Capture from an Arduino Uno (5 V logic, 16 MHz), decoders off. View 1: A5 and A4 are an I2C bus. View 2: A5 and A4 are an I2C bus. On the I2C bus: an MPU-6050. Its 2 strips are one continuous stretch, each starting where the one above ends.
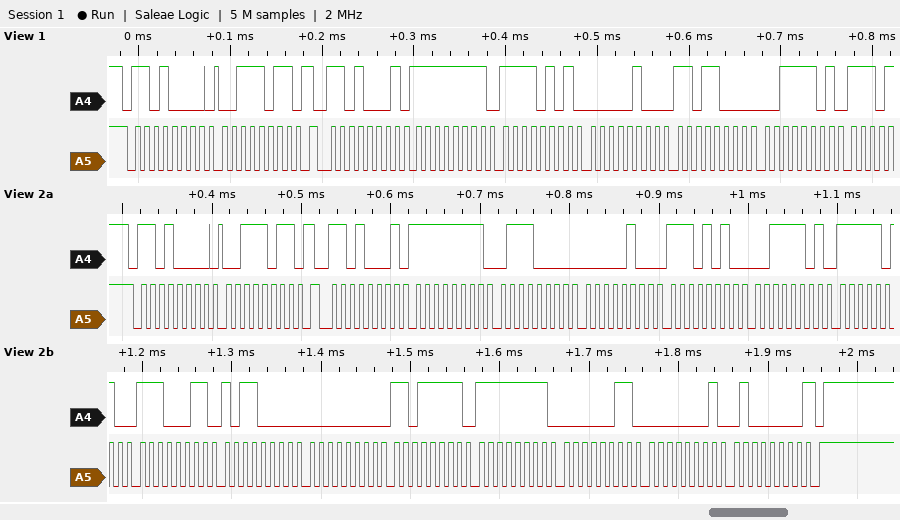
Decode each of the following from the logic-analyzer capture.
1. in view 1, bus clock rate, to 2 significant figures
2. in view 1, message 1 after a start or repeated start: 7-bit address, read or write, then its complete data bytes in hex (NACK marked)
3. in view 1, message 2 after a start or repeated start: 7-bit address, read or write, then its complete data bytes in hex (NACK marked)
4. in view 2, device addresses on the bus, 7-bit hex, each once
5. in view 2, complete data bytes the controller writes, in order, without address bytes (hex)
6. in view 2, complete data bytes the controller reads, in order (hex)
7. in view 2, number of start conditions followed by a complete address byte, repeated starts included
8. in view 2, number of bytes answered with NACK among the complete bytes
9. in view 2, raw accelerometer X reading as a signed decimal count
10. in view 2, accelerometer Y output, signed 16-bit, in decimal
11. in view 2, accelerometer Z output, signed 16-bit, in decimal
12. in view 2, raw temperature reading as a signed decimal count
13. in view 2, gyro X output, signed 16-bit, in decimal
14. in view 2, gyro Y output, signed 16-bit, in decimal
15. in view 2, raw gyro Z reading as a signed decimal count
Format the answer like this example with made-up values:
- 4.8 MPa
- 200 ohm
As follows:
- 100 kHz
- 0x68 write: 3B
- 0x68 read: FF F5 04 D8 3D
- 0x68
- 3B
- FF 70 04 EA 3D FA E3 B0 00 DF FF 03 01 40
- 2
- 1
- -144
- 1258
- 15866
- -7248
- 223
- -253
- 320
